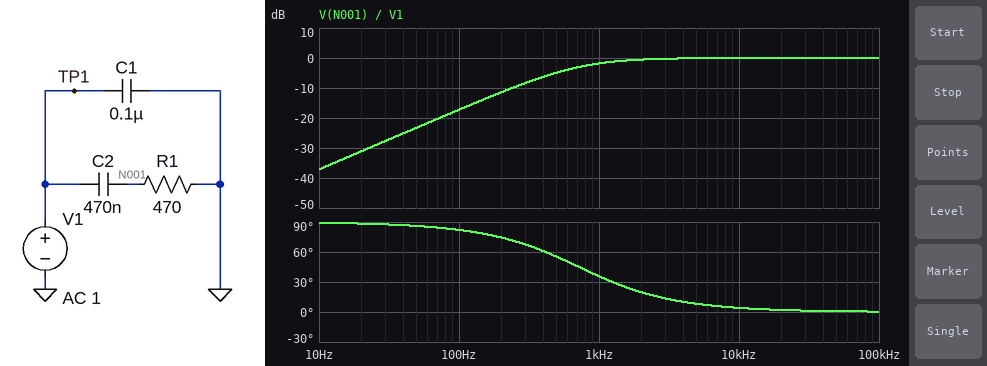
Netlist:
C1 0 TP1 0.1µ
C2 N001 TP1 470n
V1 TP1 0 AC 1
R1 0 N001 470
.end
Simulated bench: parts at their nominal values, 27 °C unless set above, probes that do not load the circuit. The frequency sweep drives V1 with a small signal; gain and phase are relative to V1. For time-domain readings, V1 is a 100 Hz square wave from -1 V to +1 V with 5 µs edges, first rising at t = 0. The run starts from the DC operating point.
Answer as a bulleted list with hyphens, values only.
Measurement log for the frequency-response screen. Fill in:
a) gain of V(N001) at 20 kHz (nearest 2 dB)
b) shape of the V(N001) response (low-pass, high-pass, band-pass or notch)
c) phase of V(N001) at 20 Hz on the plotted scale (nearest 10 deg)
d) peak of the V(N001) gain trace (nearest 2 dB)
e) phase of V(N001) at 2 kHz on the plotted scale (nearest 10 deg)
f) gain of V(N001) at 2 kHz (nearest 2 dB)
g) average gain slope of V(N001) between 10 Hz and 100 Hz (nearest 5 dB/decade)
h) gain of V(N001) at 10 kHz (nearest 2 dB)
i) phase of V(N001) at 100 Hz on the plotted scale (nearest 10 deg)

- 0 dB
- high-pass
- 90 deg
- 0 dB
- 20 deg
- 0 dB
- 20 dB/decade
- 0 dB
- 80 deg
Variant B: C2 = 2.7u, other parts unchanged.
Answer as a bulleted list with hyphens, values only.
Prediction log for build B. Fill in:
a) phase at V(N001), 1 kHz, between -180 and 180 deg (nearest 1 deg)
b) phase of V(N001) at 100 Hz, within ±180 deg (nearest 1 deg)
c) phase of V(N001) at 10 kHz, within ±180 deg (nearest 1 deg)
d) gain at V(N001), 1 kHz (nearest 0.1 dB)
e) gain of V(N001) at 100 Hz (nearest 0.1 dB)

- 7 deg
- 51 deg
- 1 deg
- -0.1 dB
- -4.1 dB
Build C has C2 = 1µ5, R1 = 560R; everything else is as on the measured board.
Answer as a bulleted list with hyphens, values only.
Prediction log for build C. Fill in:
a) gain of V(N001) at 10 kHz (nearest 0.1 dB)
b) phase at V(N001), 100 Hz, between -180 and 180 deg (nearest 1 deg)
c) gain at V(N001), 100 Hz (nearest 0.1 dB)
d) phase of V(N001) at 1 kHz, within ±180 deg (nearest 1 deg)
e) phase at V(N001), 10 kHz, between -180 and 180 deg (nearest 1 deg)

- 0 dB
- 62 deg
- -6.6 dB
- 11 deg
- 1 deg
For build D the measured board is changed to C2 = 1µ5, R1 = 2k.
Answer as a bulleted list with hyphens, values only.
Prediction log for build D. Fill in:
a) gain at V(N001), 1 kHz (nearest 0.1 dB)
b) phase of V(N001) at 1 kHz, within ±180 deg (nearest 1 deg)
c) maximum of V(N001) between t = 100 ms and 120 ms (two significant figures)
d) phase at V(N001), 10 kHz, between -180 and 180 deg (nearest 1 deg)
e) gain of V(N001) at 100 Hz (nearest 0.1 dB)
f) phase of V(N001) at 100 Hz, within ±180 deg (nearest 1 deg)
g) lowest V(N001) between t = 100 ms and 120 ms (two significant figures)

- 0 dB
- 3 deg
- 1.7 V
- 0 deg
- -1.1 dB
- 28 deg
- -1.7 V
